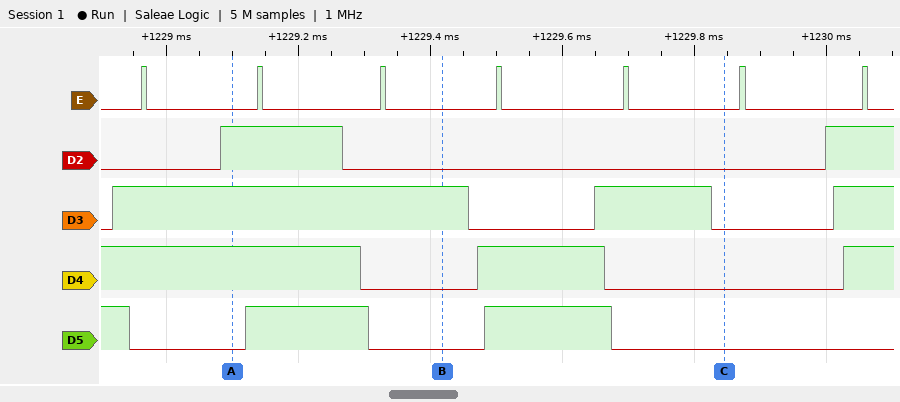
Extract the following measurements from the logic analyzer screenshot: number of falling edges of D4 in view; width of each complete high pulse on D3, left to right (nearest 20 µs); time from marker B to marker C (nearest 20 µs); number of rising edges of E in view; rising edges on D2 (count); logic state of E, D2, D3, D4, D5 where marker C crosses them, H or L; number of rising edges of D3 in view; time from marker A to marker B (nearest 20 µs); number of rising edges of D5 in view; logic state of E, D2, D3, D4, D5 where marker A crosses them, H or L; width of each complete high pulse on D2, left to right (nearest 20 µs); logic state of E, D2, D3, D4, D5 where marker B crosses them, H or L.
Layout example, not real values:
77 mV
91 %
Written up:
2
540 µs, 180 µs
420 µs
7
2
E=L, D2=L, D3=L, D4=L, D5=L
3
320 µs
2
E=L, D2=H, D3=H, D4=H, D5=L
180 µs
E=L, D2=L, D3=H, D4=L, D5=L
